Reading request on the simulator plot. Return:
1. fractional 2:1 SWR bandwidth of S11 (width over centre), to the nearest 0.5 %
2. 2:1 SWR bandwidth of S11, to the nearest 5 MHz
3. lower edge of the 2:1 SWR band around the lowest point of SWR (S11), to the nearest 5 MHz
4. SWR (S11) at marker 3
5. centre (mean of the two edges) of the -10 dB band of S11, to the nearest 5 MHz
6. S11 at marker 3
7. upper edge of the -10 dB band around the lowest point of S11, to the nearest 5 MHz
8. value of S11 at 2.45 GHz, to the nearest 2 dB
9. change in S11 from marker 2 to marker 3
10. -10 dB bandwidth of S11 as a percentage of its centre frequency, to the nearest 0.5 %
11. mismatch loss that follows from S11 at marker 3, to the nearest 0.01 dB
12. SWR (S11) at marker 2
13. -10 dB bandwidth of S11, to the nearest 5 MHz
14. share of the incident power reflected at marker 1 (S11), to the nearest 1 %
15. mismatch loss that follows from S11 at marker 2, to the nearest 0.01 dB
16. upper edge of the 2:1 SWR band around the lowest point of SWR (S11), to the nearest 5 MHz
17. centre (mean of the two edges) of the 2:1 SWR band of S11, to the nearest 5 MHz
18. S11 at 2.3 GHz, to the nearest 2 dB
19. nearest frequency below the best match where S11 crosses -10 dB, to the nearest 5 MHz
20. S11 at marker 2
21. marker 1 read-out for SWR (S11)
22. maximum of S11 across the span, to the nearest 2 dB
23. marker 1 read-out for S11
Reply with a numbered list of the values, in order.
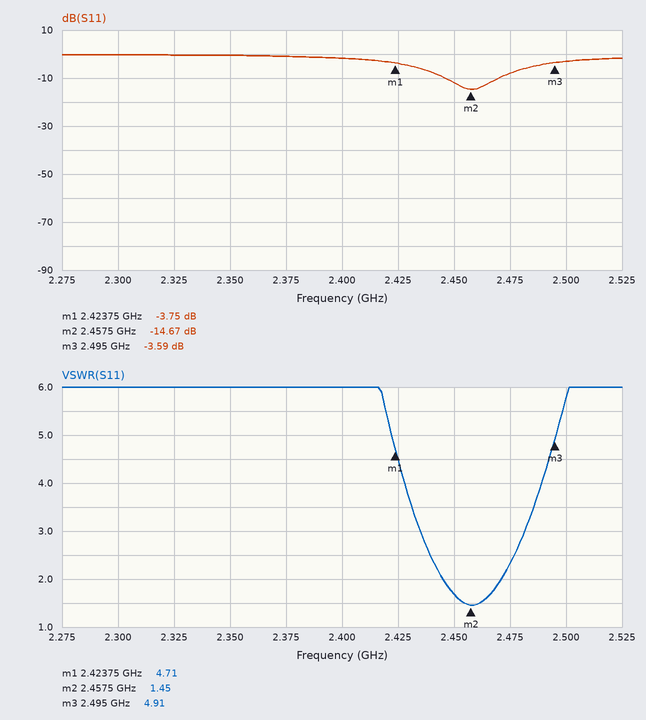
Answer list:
1. 1.0 %
2. 25 MHz
3. 2.445 GHz
4. 4.91
5. 2.460 GHz
6. -3.59 dB
7. 2.470 GHz
8. -12 dB
9. 11.08 dB
10. 1.0 %
11. 2.50 dB
12. 1.45
13. 25 MHz
14. 42 %
15. 0.15 dB
16. 2.470 GHz
17. 2.460 GHz
18. 0 dB
19. 2.445 GHz
20. -14.67 dB
21. 4.71
22. 0 dB
23. -3.75 dB
